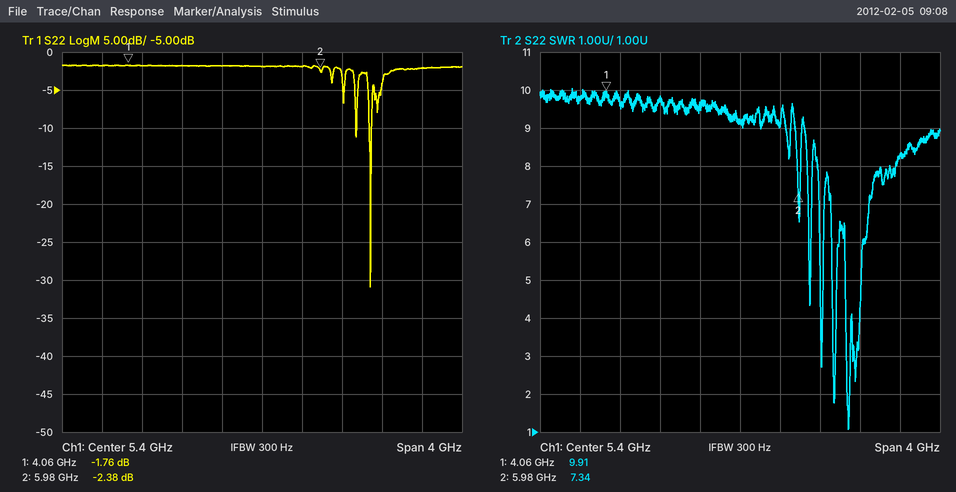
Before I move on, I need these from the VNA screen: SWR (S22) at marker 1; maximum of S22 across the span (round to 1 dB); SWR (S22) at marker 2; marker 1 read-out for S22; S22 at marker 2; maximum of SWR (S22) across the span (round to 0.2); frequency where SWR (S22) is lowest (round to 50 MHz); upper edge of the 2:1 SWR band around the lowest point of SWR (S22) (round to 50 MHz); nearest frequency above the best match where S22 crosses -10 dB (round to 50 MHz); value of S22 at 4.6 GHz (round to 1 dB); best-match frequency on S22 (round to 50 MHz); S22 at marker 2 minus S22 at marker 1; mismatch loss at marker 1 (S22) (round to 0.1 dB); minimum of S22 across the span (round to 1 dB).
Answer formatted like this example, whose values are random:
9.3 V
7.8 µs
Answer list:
9.91
-2 dB
7.34
-1.76 dB
-2.38 dB
10.0
6.50 GHz
6.50 GHz
6.50 GHz
-2 dB
6.50 GHz
-0.62 dB
4.8 dB
-31 dB
